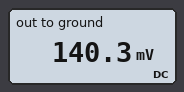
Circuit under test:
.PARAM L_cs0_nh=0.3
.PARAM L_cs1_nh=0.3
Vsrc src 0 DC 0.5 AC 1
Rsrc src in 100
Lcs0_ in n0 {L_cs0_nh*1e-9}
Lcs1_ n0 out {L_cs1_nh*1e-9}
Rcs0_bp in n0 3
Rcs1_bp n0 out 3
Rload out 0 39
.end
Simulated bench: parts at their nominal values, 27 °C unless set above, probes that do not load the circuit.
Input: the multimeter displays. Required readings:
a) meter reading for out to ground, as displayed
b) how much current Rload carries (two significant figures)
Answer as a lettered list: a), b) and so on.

a) 140.3 mV
b) 3.6 mA
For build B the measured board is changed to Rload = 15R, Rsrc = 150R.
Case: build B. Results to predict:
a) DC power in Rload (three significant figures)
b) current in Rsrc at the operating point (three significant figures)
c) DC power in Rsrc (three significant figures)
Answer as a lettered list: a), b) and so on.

a) 138 µW
b) 3.03 mA
c) 1.38 mW
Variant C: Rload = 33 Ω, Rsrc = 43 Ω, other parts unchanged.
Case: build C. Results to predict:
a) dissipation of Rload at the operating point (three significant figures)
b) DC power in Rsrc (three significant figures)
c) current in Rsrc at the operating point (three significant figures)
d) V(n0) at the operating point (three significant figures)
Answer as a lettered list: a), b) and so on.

a) 1.43 mW
b) 1.86 mW
c) 6.58 mA
d) 217 mV
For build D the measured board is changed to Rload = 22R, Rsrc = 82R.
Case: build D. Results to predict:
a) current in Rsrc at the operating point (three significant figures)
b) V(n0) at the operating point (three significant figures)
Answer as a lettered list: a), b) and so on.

a) 4.81 mA
b) 106 mV
